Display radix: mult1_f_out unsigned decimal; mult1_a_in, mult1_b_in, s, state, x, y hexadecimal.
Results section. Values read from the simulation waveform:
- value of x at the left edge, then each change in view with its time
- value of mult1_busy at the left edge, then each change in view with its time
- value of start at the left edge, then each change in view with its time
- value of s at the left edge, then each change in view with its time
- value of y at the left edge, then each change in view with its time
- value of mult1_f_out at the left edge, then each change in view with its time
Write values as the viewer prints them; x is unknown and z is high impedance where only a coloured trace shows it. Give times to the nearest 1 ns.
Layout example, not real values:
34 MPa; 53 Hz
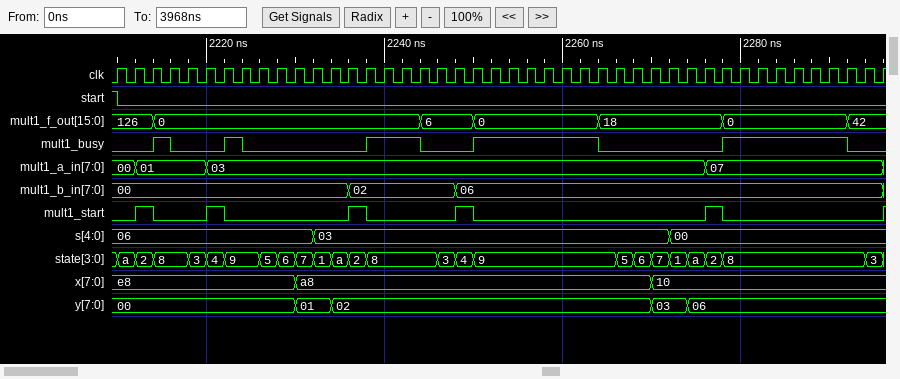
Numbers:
e8, a8 at 2230 ns, 10 at 2270 ns; 0, 1 at 2214 ns, 0 at 2216 ns, 1 at 2222 ns, 0 at 2224 ns, 1 at 2238 ns, 0 at 2244 ns, 1 at 2250 ns, 0 at 2264 ns, 1 at 2278 ns, 0 at 2292 ns; 1, 0 at 2210 ns; 06, 03 at 2232 ns, 00 at 2272 ns; 00, 01 at 2230 ns, 02 at 2234 ns, 03 at 2270 ns, 06 at 2274 ns; 126, 0 at 2214 ns, 6 at 2244 ns, 0 at 2250 ns, 18 at 2264 ns, 0 at 2278 ns, 42 at 2292 ns
